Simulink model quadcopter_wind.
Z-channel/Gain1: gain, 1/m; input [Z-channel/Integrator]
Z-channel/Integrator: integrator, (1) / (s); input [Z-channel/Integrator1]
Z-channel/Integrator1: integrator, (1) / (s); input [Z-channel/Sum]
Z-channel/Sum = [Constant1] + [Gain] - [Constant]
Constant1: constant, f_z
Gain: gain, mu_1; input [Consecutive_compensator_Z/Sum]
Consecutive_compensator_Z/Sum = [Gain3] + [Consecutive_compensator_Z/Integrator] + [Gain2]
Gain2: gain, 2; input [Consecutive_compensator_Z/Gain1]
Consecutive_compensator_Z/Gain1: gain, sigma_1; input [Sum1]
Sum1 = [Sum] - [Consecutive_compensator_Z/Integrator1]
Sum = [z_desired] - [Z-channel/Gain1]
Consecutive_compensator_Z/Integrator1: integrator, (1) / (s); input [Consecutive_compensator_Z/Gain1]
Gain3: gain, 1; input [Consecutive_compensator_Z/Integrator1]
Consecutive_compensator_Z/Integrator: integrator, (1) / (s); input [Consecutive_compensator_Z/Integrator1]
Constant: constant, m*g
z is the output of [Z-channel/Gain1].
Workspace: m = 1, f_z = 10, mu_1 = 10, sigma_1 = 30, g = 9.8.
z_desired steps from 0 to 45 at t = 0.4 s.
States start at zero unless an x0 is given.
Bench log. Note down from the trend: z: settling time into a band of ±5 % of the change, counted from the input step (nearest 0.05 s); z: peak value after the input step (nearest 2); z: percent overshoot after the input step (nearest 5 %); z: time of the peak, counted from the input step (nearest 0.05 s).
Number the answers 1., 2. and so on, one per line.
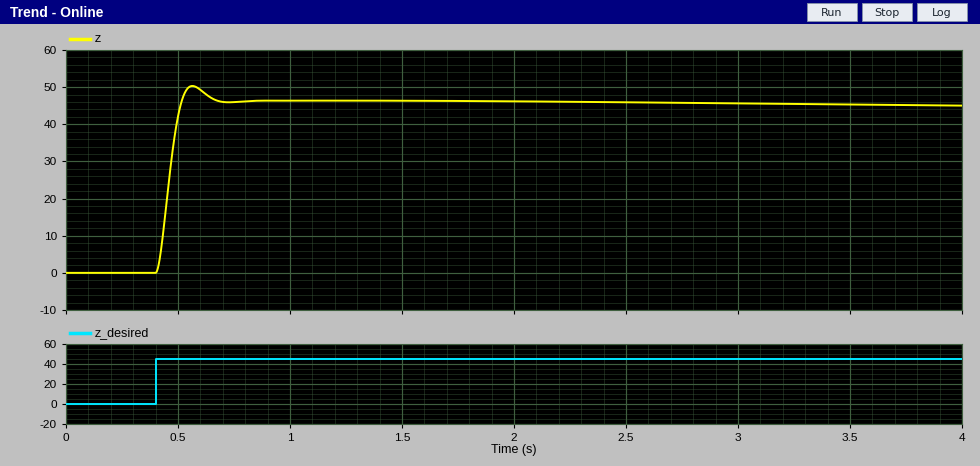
1. 0.25 s
2. 50
3. 10 %
4. 0.15 s
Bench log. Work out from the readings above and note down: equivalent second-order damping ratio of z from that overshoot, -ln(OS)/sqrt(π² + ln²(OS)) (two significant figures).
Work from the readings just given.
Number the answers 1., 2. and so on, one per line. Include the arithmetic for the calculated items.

1. ln(0.1) = -2.303; 2.303 / sqrt(9.870 + 5.302) = 0.59
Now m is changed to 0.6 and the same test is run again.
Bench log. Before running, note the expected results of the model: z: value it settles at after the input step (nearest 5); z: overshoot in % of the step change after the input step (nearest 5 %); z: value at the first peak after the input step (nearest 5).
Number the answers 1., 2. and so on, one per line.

1. 45
2. 20 %
3. 55
